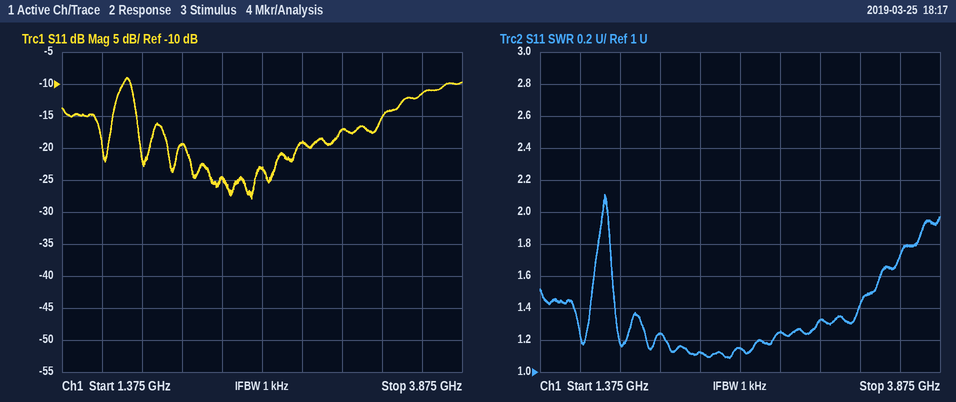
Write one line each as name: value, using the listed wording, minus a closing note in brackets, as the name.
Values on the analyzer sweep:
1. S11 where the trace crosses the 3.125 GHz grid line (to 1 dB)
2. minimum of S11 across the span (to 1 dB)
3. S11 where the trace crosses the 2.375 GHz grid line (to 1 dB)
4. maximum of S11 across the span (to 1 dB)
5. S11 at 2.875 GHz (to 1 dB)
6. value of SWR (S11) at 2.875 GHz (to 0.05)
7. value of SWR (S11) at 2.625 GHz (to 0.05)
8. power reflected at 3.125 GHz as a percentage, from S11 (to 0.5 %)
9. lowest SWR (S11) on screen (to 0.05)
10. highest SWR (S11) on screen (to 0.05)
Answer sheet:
S11 where the trace crosses the 3.125 GHz grid line: -17 dB
minimum of S11 across the span: -28 dB
S11 where the trace crosses the 2.375 GHz grid line: -25 dB
maximum of S11 across the span: -9 dB
S11 at 2.875 GHz: -19 dB
value of SWR (S11) at 2.875 GHz: 1.25
value of SWR (S11) at 2.625 GHz: 1.15
power reflected at 3.125 GHz as a percentage, from S11: 2.0 %
lowest SWR (S11) on screen: 1.10
highest SWR (S11) on screen: 2.10
